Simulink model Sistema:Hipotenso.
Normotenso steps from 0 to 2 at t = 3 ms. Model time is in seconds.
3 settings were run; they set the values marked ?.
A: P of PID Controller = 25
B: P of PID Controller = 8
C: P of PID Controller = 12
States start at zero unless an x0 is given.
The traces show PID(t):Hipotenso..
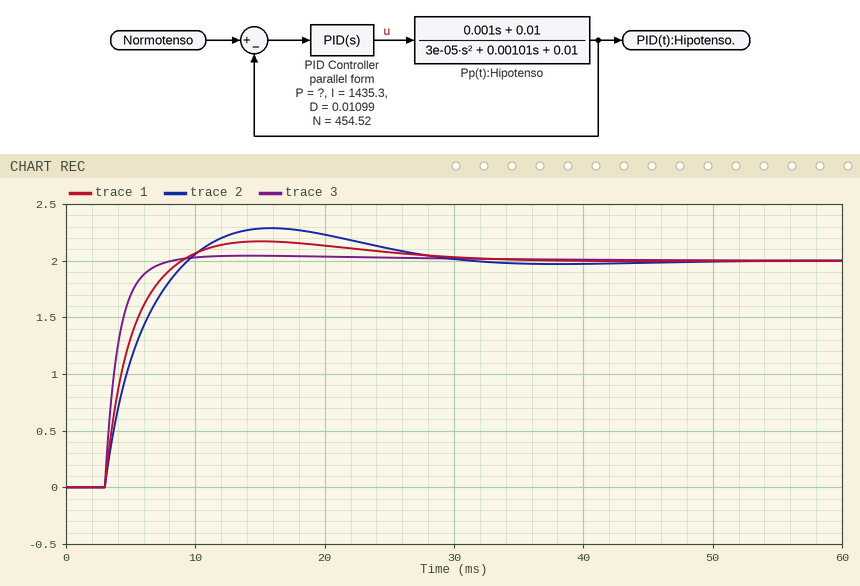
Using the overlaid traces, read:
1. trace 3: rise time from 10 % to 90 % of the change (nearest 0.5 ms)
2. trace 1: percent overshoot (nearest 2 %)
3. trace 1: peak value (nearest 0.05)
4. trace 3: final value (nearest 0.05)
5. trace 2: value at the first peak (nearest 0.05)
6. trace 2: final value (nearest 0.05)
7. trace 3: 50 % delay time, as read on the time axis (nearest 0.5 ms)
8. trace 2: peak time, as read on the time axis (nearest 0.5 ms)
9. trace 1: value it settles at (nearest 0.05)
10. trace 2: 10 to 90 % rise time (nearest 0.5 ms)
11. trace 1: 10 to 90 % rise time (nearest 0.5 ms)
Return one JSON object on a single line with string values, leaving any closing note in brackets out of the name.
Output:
{"trace 3: rise time from 10 % to 90 % of the change": "2.5 ms", "trace 1: percent overshoot": "8 %", "trace 1: peak value": "2.15", "trace 3: final value": "2.00", "trace 2: value at the first peak": "2.30", "trace 2: final value": "2.00", "trace 3: 50 % delay time, as read on the time axis": "3.5 ms", "trace 2: peak time, as read on the time axis": "16.0 ms", "trace 1: value it settles at": "2.00", "trace 2: 10 to 90 % rise time": "4.5 ms", "trace 1: 10 to 90 % rise time": "4.0 ms"}
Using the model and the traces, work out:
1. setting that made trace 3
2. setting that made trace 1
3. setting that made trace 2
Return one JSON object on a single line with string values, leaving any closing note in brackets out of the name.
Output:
{"setting that made trace 3": "A", "setting that made trace 1": "C", "setting that made trace 2": "B"}
